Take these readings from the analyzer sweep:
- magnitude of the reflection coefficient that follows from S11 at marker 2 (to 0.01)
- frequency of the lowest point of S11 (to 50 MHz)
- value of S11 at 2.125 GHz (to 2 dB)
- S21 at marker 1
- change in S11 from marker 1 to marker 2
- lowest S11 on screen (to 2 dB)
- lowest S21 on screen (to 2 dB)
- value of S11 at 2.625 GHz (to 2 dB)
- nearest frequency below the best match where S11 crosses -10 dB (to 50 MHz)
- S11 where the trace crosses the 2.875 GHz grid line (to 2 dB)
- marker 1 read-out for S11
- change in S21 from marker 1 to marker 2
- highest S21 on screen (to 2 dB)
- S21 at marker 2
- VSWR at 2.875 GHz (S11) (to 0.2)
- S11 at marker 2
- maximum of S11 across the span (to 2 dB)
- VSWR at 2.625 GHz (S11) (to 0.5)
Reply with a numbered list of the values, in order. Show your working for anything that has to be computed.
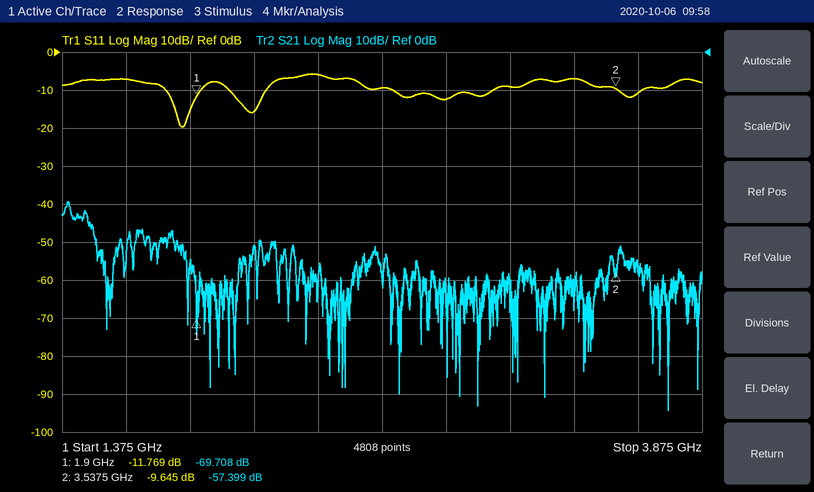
1. 10^(-9.645/20) ≈ 0.33
2. 1.85 GHz
3. -16 dB
4. -69.708 dB
5. -9.645 − (-11.769) = 2.124 dB
6. -20 dB
7. -94 dB
8. -10 dB
9. 1.80 GHz
10. -12 dB
11. -11.769 dB
12. -57.399 − (-69.708) = 12.309 dB
13. -40 dB
14. -57.399 dB
15. |Γ| = 10^(-12/20) = 0.2512; VSWR = (1 + 0.2512)/(1 − 0.2512) ≈ 1.67, so 1.6 to the nearest 0.2
16. -9.645 dB
17. -6 dB
18. |Γ| = 10^(-10/20) = 0.3162; VSWR = (1 + 0.3162)/(1 − 0.3162) ≈ 1.92, so 2.0 to the nearest 0.5
